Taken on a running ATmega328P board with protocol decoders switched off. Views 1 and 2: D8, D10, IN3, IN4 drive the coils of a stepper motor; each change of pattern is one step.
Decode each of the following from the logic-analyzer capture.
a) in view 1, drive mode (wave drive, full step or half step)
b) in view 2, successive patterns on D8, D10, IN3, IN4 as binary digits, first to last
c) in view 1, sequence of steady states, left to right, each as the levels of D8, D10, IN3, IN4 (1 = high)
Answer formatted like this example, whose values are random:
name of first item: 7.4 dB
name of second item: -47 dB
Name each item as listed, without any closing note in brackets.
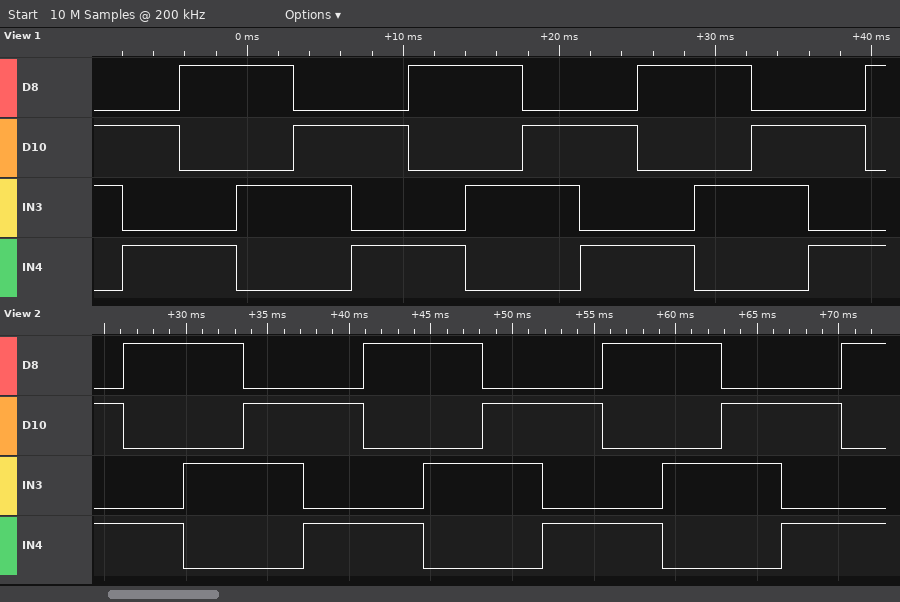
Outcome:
in view 1, drive mode: full step
in view 2, successive patterns on D8, D10, IN3, IN4 as binary digits, first to last: 0101 1001 1010 0110 0101 1001 1010 0110 0101 1001 1010 0110 0101 1001
in view 1, sequence of steady states, left to right, each as the levels of D8, D10, IN3, IN4: 0110 0101 1001 1010 0110 0101 1001 1010 0110 0101 1001 1010 0110 0101 1001
